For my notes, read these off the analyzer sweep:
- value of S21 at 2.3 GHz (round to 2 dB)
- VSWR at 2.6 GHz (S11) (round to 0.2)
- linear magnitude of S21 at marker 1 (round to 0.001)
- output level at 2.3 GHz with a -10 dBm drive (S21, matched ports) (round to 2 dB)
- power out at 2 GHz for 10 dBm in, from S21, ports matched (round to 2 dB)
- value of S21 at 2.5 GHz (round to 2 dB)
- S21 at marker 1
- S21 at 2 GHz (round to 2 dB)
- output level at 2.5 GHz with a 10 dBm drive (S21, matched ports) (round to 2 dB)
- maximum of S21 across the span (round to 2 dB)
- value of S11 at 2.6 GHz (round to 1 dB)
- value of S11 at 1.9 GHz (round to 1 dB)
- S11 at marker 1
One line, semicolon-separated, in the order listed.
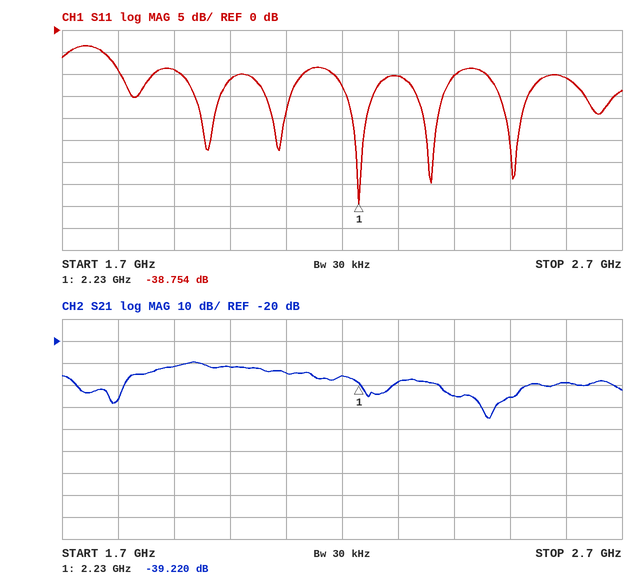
-38 dB; 1.8; 0.011; -48 dBm; -22 dBm; -46 dB; -39.220 dB; -32 dB; -36 dBm; -30 dB; -11 dB; -9 dB; -38.754 dB
